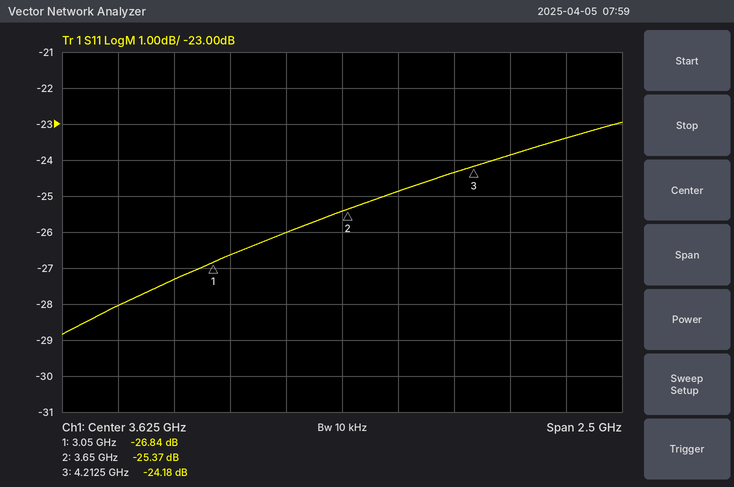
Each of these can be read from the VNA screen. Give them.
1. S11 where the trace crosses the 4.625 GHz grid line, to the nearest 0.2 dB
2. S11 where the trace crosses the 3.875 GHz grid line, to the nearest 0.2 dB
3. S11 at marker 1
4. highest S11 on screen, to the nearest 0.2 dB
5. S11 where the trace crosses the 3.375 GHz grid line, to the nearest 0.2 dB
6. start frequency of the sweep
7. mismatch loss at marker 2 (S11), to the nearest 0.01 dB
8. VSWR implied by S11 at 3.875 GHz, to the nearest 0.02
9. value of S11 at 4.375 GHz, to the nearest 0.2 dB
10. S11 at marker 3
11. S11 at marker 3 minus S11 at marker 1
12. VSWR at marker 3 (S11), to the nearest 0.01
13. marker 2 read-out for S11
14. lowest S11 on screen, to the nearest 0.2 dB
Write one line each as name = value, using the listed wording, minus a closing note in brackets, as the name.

S11 where the trace crosses the 4.625 GHz grid line, to the nearest 0.2 dB = -23.4 dB
S11 where the trace crosses the 3.875 GHz grid line, to the nearest 0.2 dB = -24.8 dB
S11 at marker 1 = -26.84 dB
highest S11 on screen, to the nearest 0.2 dB = -23.0 dB
S11 where the trace crosses the 3.375 GHz grid line, to the nearest 0.2 dB = -26.0 dB
start frequency of the sweep = 2.375 GHz
mismatch loss at marker 2 (S11), to the nearest 0.01 dB = 0.01 dB
VSWR implied by S11 at 3.875 GHz, to the nearest 0.02 = 1.12
value of S11 at 4.375 GHz, to the nearest 0.2 dB = -23.8 dB
S11 at marker 3 = -24.18 dB
S11 at marker 3 minus S11 at marker 1 = 2.66 dB
VSWR at marker 3 (S11), to the nearest 0.01 = 1.13
marker 2 read-out for S11 = -25.37 dB
lowest S11 on screen, to the nearest 0.2 dB = -28.8 dB
